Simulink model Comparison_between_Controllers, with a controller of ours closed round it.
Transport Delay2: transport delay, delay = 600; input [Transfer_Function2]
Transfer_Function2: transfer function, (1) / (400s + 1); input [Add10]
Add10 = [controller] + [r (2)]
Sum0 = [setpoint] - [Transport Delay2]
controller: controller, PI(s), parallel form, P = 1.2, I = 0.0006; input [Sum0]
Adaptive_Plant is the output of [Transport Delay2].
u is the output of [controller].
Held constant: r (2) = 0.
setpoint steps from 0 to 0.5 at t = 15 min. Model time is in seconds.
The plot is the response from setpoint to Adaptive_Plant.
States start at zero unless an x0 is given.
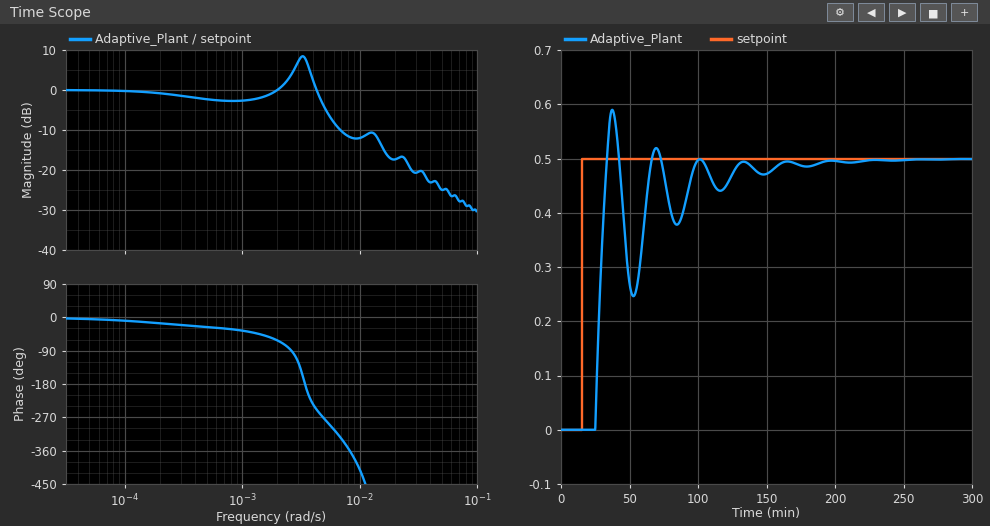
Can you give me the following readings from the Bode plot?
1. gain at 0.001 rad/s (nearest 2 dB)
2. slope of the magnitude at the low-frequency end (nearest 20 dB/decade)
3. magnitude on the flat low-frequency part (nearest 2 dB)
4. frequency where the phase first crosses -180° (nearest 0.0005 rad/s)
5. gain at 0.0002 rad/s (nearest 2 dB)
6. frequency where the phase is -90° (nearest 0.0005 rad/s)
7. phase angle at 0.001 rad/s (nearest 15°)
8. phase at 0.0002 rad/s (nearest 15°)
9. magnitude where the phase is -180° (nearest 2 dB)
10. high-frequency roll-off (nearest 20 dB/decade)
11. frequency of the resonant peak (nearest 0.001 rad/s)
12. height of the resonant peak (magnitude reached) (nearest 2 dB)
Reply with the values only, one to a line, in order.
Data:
-2 dB
0 dB/decade
0 dB
0.0035 rad/s
0 dB
0.0025 rad/s
-30°
-15°
8 dB
-20 dB/decade
0.003 rad/s
8 dB
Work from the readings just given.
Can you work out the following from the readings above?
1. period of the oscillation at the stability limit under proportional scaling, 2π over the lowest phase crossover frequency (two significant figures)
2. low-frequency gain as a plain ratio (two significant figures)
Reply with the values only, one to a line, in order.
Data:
1800 s
1.0
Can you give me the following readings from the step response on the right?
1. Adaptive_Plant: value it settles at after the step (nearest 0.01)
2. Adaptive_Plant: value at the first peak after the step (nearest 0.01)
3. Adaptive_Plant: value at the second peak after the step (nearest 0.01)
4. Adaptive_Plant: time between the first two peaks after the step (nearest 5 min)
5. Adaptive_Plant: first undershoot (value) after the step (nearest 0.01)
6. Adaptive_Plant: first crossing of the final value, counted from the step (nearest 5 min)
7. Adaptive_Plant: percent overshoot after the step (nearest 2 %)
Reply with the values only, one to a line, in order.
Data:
0.50
0.59
0.52
30 min
0.25
20 min
18 %
